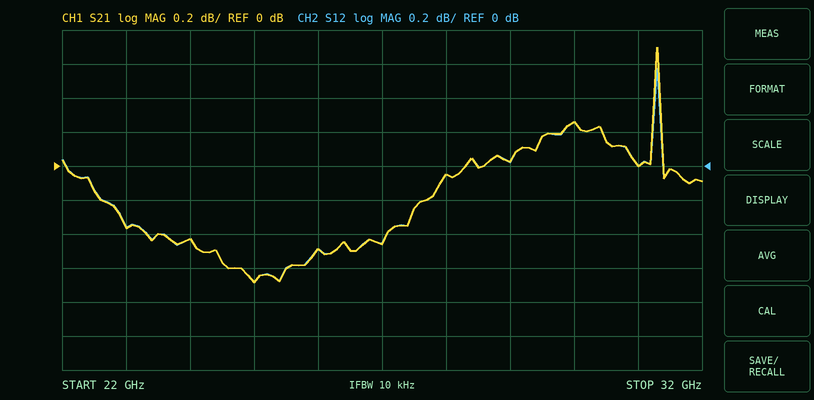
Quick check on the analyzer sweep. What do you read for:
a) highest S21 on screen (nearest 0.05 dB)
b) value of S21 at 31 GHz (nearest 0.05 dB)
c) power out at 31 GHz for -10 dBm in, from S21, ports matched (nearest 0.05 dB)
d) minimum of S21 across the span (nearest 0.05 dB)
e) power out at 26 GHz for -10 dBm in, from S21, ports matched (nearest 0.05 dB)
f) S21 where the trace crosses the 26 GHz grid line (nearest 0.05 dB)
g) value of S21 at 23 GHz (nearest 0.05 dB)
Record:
0.70 dB
0.00 dB
-10.00 dBm
-0.70 dB
-10.50 dBm
-0.50 dB
-0.35 dB
